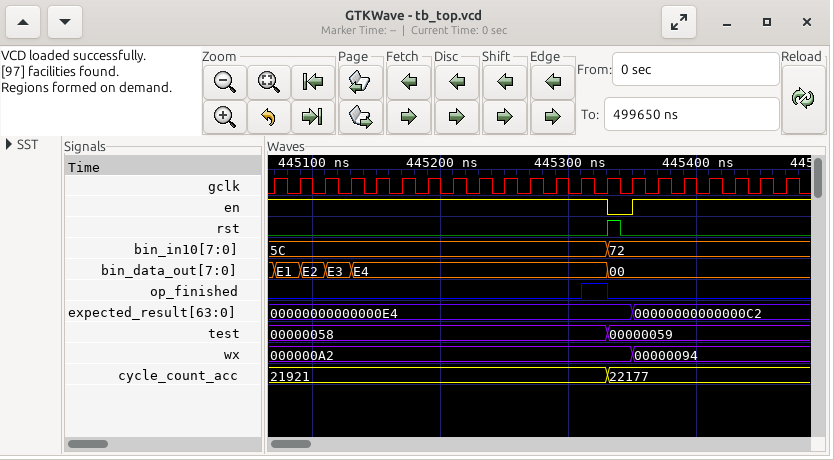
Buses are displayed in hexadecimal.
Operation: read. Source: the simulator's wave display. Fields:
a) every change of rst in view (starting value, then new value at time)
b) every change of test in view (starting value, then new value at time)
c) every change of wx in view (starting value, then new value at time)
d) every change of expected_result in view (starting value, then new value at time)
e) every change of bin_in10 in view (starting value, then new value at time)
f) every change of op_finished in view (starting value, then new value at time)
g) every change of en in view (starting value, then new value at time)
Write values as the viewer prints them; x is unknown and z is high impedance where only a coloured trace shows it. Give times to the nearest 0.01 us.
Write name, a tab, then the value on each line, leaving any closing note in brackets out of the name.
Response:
every change of rst in view	0, 1 at 445.33 us, 0 at 445.34 us
every change of test in view	00000058, 00000059 at 445.33 us
every change of wx in view	000000A2, 00000094 at 445.35 us
every change of expected_result in view	00000000000000E4, 00000000000000C2 at 445.35 us
every change of bin_in10 in view	5C, 72 at 445.33 us
every change of op_finished in view	0, 1 at 445.31 us, 0 at 445.33 us
every change of en in view	1, 0 at 445.33 us, 1 at 445.35 us
